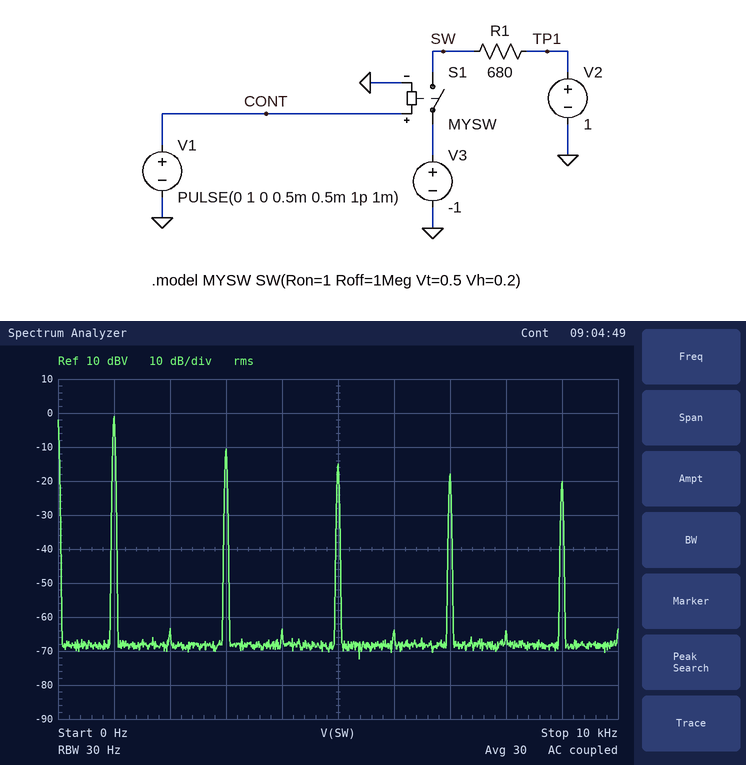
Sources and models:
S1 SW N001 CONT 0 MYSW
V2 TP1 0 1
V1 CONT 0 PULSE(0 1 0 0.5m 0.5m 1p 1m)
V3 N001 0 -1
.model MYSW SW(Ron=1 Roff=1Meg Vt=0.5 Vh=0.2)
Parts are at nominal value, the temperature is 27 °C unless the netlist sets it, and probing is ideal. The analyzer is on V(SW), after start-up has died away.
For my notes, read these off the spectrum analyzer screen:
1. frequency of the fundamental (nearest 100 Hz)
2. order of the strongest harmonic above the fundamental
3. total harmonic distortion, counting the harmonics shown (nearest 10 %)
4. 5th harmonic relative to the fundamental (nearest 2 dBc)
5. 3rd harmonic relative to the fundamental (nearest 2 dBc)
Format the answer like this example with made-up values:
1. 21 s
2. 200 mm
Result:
1. 1.0 kHz
2. 3
3. 40 %
4. -14 dBc
5. -10 dBc
